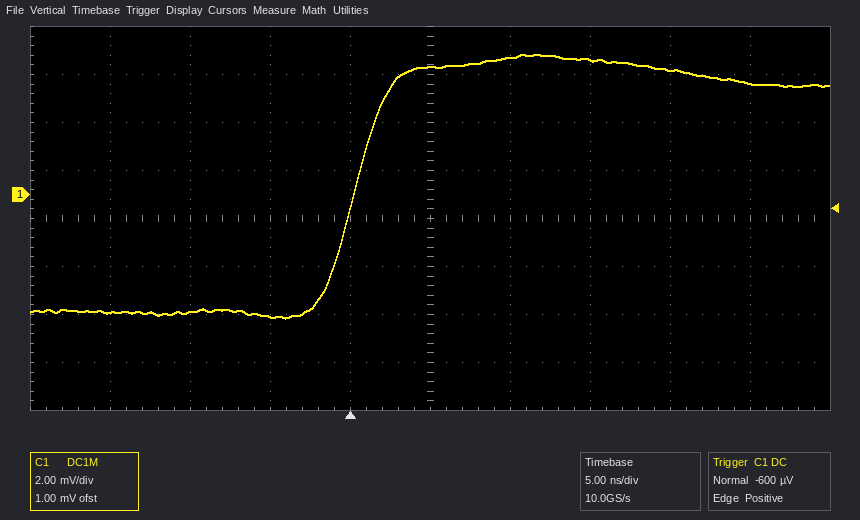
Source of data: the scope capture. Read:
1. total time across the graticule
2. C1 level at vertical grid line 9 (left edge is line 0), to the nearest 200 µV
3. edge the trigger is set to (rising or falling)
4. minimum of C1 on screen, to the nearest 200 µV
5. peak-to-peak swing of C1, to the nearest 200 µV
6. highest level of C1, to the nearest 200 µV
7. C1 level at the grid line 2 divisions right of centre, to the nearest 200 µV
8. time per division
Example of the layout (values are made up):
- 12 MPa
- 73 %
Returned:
- 50 ns
- 4.6 mV
- rising
- -5.2 mV
- 11.0 mV
- 5.8 mV
- 5.6 mV
- 5 ns
